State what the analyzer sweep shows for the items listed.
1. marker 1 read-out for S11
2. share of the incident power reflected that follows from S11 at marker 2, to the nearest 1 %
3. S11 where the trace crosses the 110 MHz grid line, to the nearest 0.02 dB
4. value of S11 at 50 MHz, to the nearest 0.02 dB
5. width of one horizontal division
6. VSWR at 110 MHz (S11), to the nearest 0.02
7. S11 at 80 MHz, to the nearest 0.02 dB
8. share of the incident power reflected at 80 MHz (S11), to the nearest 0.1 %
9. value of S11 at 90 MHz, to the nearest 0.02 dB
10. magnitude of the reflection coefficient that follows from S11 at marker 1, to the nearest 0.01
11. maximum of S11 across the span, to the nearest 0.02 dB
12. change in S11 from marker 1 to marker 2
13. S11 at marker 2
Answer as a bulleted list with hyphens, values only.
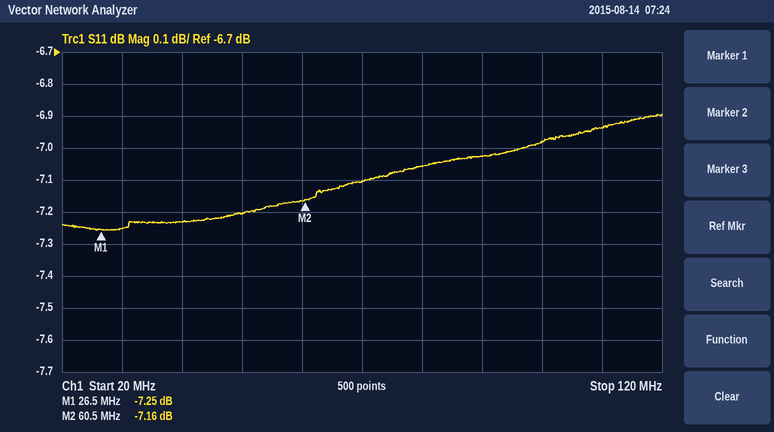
- -7.25 dB
- 19 %
- -6.94 dB
- -7.20 dB
- 10 MHz
- 2.64
- -7.06 dB
- 19.7 %
- -7.02 dB
- 0.43
- -6.90 dB
- 0.09 dB
- -7.16 dB
